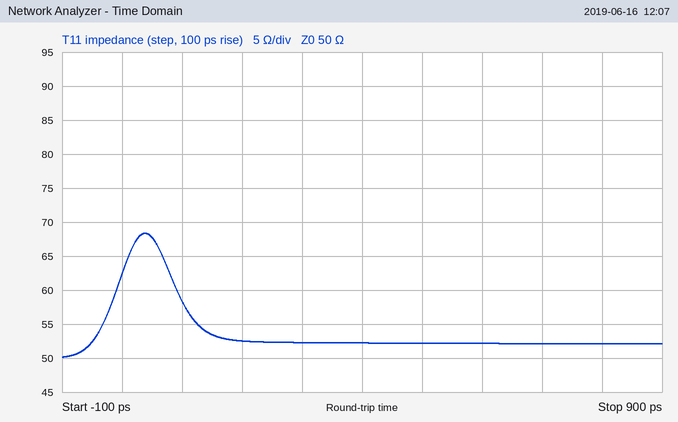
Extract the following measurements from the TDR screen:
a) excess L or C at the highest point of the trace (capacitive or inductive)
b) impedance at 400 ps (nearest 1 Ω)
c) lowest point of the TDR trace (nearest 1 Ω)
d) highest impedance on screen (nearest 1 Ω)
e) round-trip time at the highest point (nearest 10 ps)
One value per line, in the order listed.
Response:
inductive
52 Ω
50 Ω
68 Ω
40 ps
